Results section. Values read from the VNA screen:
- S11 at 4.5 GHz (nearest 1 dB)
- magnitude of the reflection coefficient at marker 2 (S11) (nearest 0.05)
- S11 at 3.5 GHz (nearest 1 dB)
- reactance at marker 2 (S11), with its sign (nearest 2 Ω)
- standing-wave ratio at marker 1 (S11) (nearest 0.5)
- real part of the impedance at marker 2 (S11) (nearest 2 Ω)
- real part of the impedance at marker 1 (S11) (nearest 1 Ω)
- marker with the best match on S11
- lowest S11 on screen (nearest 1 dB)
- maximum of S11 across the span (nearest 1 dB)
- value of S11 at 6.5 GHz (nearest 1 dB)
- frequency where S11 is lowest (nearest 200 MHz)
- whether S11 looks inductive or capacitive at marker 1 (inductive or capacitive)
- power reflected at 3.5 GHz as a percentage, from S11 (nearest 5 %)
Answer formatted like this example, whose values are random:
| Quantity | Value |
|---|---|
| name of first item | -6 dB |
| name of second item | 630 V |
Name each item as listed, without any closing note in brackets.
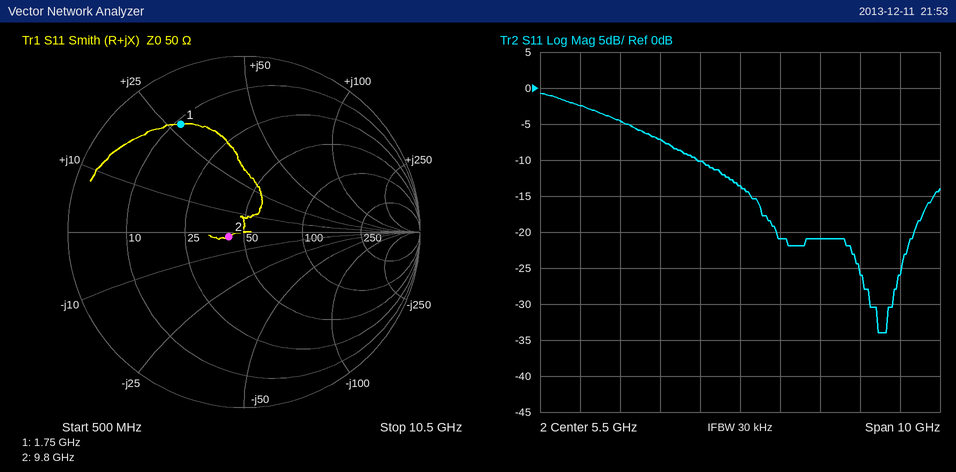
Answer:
| Quantity | Value |
|---|---|
| S11 at 4.5 GHz | -10 dB |
| magnitude of the reflection coefficient at marker 2 (S11) | 0.10 |
| S11 at 3.5 GHz | -7 dB |
| reactance at marker 2 (S11), with its sign | -2 Ω |
| standing-wave ratio at marker 1 (S11) | 6.0 |
| real part of the impedance at marker 2 (S11) | 42 Ω |
| real part of the impedance at marker 1 (S11) | 11 Ω |
| marker with the best match on S11 | marker 2 |
| lowest S11 on screen | -34 dB |
| maximum of S11 across the span | -1 dB |
| value of S11 at 6.5 GHz | -21 dB |
| frequency where S11 is lowest | 9.0 GHz |
| whether S11 looks inductive or capacitive at marker 1 | inductive |
| power reflected at 3.5 GHz as a percentage, from S11 | 20 % |
